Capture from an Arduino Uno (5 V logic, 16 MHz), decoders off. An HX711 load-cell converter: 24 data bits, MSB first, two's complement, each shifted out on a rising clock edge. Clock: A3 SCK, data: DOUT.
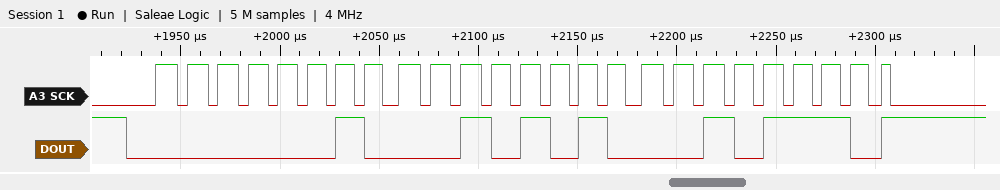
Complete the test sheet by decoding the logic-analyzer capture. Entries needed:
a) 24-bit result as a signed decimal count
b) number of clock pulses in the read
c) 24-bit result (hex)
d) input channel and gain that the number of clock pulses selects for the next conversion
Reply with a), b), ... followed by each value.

a) 141870
b) 25
c) 0x022A2E
d) channel A, gain 128
